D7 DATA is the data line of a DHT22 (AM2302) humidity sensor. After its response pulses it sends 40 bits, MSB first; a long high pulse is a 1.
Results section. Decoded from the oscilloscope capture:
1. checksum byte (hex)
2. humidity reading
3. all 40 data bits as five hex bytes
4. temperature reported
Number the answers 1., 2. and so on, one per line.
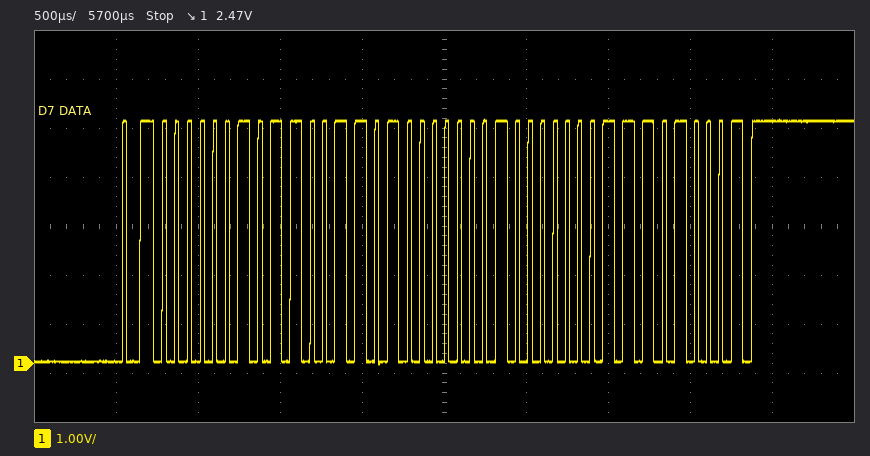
1. 0xD1
2. 71.7 %
3. 02 CD 01 01 D1
4. 25.7 °C
